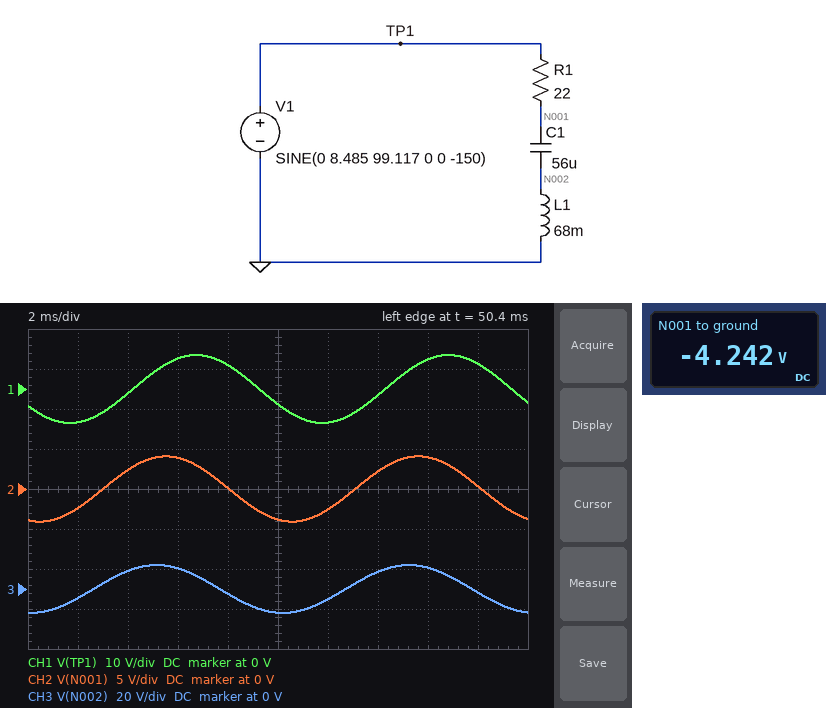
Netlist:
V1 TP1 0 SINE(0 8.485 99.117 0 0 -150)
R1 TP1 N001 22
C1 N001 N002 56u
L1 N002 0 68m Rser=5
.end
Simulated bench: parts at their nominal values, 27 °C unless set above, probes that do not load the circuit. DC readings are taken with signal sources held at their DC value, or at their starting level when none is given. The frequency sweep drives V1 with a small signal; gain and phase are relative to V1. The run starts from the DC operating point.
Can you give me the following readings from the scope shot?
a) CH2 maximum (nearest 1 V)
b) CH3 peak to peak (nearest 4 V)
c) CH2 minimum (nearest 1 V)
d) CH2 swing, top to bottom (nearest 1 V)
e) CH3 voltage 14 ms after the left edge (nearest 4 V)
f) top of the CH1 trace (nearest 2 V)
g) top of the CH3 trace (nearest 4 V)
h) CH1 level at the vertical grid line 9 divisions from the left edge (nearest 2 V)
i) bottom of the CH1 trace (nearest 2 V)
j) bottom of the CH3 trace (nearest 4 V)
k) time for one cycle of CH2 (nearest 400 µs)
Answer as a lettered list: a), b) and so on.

a) 4 V
b) 24 V
c) -4 V
d) 8 V
e) 8 V
f) 8 V
g) 12 V
h) 6 V
i) -8 V
j) -12 V
k) 10.0 ms
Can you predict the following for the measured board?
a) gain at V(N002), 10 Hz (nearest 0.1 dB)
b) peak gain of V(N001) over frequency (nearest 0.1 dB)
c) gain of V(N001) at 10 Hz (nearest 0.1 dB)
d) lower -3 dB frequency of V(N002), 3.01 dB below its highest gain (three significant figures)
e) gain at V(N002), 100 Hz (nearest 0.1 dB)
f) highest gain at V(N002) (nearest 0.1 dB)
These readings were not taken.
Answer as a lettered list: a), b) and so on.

a) -32.6 dB
b) 0 dB
c) 0 dB
d) 68.3 Hz
e) 3.0 dB
f) 3.0 dB
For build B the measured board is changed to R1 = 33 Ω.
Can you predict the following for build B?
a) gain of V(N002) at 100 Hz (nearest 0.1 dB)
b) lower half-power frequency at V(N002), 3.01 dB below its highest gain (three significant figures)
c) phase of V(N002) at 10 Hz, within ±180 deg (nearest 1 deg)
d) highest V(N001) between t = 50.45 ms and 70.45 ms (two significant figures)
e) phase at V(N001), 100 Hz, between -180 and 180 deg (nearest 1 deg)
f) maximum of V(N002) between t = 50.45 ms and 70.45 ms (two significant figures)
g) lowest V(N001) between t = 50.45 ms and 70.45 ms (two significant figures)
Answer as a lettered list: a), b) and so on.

a) 0.5 dB
b) 70.5 Hz
c) 123 deg
d) 3.1 V
e) 50 deg
f) 9.0 V
g) -3.1 V
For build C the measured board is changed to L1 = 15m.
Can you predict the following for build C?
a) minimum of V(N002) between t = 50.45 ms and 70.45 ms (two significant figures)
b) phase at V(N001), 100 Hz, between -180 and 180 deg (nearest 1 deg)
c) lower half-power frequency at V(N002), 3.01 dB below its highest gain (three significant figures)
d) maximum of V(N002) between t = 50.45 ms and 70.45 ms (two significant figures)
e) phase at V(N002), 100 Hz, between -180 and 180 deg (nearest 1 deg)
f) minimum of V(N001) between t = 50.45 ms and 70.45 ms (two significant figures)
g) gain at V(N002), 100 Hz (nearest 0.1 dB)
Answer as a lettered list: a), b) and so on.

a) -2.7 V
b) -40 deg
c) 198 Hz
d) 2.7 V
e) 97 deg
f) -5.1 V
g) -9.8 dB
